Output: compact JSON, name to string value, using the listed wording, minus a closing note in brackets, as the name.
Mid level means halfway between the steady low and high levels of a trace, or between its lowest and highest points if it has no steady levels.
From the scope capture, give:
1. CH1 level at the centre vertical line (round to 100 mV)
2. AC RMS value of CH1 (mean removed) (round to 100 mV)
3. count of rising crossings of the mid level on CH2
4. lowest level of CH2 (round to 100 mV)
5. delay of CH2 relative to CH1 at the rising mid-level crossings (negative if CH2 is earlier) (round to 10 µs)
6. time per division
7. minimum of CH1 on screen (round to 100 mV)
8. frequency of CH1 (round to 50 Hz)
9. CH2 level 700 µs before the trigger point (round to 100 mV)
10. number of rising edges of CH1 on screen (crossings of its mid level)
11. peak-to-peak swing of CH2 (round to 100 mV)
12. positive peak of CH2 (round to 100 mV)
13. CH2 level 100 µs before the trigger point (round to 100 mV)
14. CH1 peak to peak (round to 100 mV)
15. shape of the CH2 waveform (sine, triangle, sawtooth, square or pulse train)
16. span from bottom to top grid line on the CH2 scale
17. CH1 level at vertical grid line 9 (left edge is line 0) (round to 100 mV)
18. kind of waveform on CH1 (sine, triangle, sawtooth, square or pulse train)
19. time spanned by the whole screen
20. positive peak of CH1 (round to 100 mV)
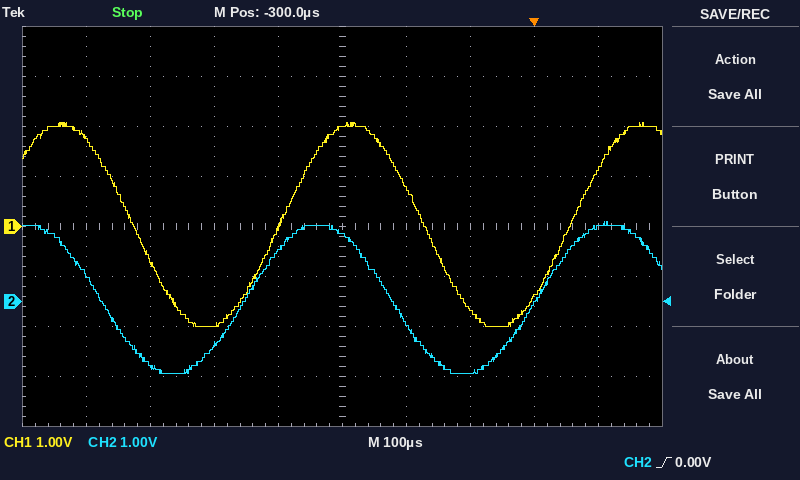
{"CH1 level at the centre vertical line": "2.0 V", "AC RMS value of CH1 (mean removed)": "1.4 V", "count of rising crossings of the mid level on CH2": "2", "lowest level of CH2": "-1.4 V", "delay of CH2 relative to CH1 at the rising mid-level crossings (negative if CH2 is earlier)": "-50 µs", "time per division": "100 µs", "minimum of CH1 on screen": "-2.0 V", "frequency of CH1": "2.20 kHz", "CH2 level 700 µs before the trigger point": "600 mV", "number of rising edges of CH1 on screen": "2", "peak-to-peak swing of CH2": "3.0 V", "positive peak of CH2": "1.6 V", "CH2 level 100 µs before the trigger point": "-1.4 V", "CH1 peak to peak": "4.1 V", "shape of the CH2 waveform": "sine", "span from bottom to top grid line on the CH2 scale": "8 V", "CH1 level at vertical grid line 9 (left edge is line 0)": "1.1 V", "kind of waveform on CH1": "sine", "time spanned by the whole screen": "1 ms", "positive peak of CH1": "2.1 V"}
